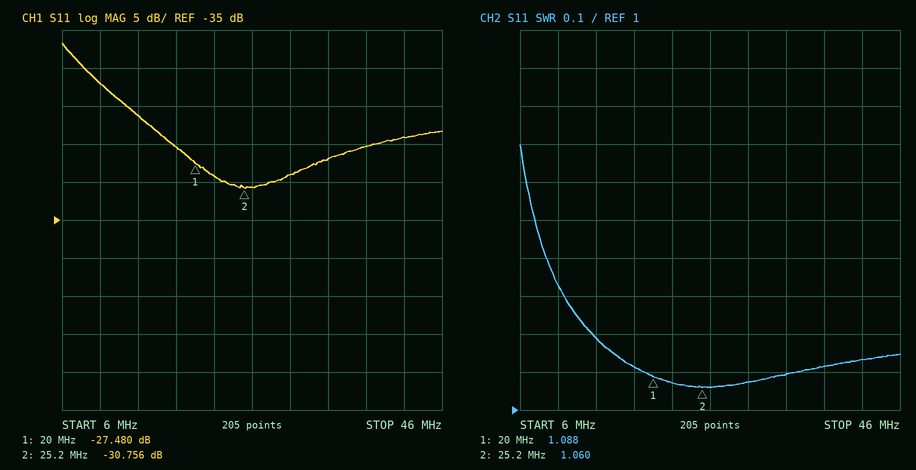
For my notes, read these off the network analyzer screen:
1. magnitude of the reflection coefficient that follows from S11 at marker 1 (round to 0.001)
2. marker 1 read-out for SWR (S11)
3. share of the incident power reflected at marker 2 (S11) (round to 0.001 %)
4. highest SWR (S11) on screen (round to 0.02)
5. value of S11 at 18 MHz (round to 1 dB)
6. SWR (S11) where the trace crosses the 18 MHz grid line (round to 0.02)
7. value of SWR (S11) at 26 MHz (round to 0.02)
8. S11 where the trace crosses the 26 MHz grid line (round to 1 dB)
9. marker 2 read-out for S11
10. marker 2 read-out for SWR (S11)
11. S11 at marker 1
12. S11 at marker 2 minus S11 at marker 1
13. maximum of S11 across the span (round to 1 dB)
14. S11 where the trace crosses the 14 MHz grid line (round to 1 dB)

0.042
1.088
0.084 %
1.70
-25 dB
1.12
1.06
-31 dB
-30.756 dB
1.060
-27.480 dB
-3.276 dB
-12 dB
-21 dB
